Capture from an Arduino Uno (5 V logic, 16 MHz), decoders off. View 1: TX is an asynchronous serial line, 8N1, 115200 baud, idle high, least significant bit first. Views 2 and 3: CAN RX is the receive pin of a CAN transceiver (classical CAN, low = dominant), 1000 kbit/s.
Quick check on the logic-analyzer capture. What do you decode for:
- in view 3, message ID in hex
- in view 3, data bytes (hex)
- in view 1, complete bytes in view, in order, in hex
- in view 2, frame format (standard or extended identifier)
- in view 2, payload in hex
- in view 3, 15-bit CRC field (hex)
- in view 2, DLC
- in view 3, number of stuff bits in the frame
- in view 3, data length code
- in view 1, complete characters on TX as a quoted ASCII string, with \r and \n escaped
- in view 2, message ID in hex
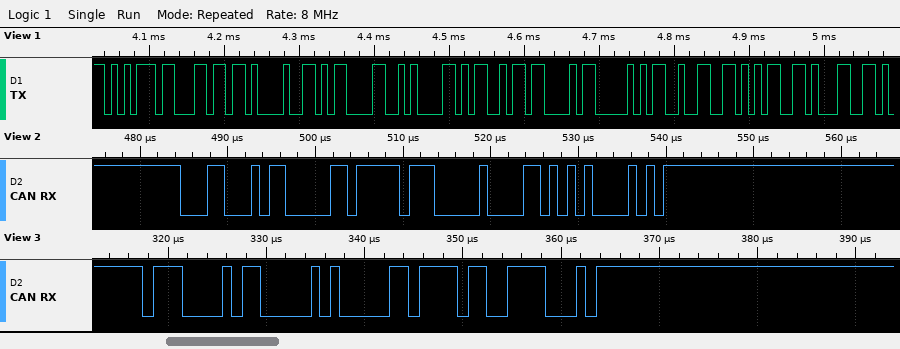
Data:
0x70B
05
0x75 0x6C 0x21 0x0D 0x0A 0x4D 0x43 0x50 0x32 0x35 0x31
standard
FF 00
0x7678
2
2
1
"ul!\r\nMCP251"
0x18B
